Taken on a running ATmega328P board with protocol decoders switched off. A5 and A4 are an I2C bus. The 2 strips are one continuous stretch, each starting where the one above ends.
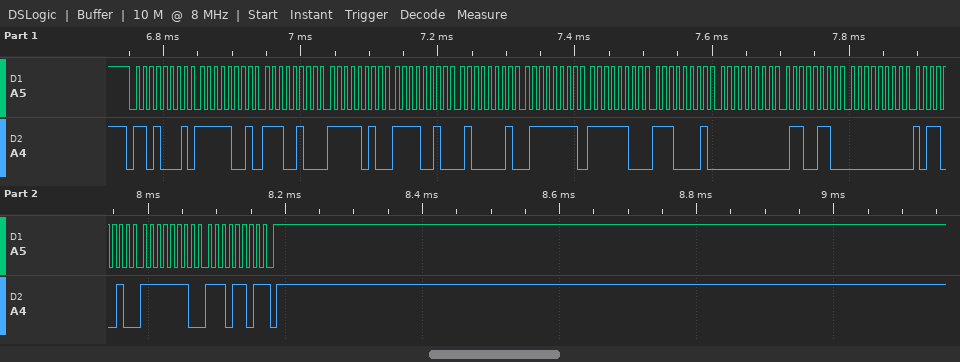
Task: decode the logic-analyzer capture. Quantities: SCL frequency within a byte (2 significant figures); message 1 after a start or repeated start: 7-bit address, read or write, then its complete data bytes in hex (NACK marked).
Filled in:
100 kHz
0x68 read: F9 E4 FA F2 41 7F FC E1 00 66 00 B2 FE ED NACK
